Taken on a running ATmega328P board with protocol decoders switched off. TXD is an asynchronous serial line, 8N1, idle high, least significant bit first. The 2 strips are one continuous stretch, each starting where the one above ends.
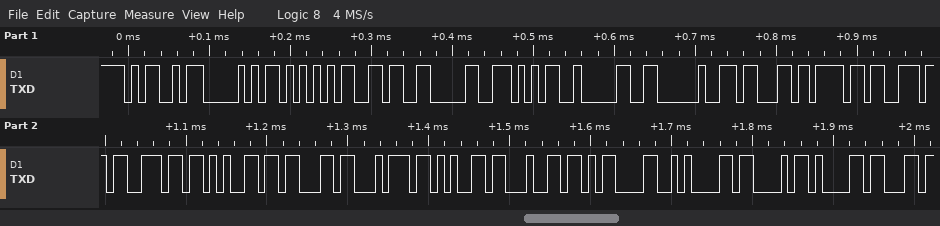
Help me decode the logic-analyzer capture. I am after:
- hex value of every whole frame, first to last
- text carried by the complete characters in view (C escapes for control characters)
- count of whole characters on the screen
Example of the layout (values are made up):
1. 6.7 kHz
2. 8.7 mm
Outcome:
1. 4D 50 55 36 30 35 30 20 63 6F 6E 6E 65 63 74 65 64 0D 0A 43 61
2. "MPU6050 connected\r\nCa"
3. 21
